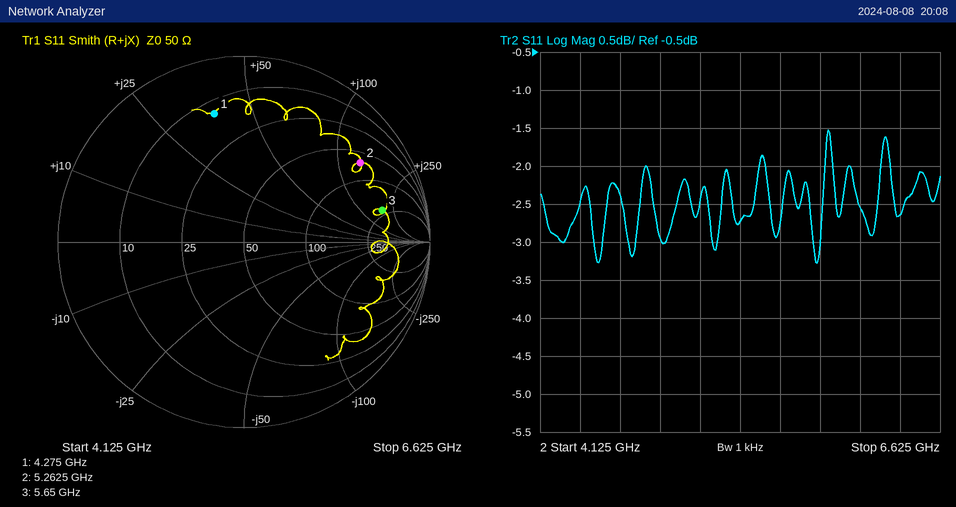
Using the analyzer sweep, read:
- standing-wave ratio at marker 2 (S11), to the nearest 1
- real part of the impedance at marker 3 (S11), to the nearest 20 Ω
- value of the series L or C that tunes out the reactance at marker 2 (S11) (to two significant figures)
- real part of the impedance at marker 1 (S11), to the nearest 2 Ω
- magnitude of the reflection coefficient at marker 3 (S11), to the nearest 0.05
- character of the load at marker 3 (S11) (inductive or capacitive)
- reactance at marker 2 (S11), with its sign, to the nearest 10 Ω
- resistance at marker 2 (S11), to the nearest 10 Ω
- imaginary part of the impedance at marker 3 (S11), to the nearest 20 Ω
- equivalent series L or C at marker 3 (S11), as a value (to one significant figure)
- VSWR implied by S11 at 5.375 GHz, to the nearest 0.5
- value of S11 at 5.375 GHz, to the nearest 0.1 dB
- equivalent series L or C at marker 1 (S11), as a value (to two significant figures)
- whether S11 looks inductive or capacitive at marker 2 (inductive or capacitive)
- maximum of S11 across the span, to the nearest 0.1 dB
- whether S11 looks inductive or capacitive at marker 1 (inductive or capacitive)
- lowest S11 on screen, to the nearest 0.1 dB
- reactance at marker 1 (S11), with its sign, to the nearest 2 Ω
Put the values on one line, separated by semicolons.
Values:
7; 220 Ω; 230 fF; 14 Ω; 0.75; inductive; +130 Ω; 70 Ω; +180 Ω; 5 nH; 6.5; -2.7 dB; 1.4 nH; inductive; -1.5 dB; inductive; -3.3 dB; +38 Ω
